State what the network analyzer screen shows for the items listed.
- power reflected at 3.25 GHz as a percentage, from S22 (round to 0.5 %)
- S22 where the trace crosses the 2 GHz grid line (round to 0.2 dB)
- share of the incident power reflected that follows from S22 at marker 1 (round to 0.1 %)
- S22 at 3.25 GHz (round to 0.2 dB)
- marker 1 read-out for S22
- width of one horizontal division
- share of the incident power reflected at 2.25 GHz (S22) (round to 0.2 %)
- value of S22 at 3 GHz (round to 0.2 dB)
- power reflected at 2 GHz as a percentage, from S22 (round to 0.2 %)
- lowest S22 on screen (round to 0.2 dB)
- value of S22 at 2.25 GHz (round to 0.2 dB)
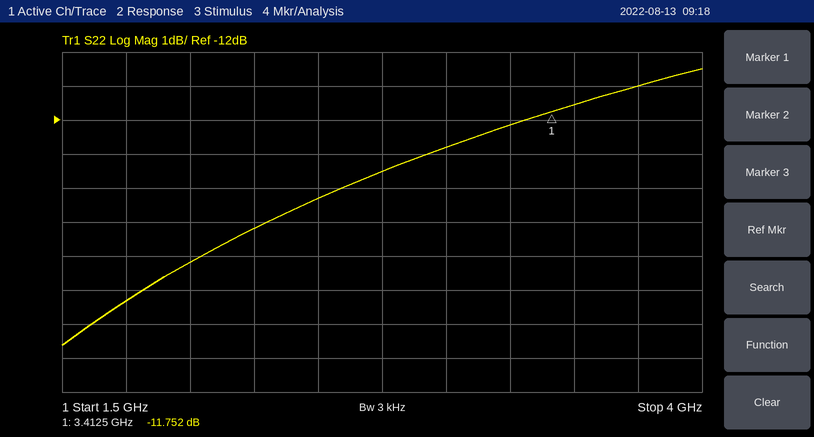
6.0 %
-16.2 dB
6.7 %
-12.2 dB
-11.752 dB
250 MHz
3.0 %
-12.8 dB
2.4 %
-18.6 dB
-15.2 dB
